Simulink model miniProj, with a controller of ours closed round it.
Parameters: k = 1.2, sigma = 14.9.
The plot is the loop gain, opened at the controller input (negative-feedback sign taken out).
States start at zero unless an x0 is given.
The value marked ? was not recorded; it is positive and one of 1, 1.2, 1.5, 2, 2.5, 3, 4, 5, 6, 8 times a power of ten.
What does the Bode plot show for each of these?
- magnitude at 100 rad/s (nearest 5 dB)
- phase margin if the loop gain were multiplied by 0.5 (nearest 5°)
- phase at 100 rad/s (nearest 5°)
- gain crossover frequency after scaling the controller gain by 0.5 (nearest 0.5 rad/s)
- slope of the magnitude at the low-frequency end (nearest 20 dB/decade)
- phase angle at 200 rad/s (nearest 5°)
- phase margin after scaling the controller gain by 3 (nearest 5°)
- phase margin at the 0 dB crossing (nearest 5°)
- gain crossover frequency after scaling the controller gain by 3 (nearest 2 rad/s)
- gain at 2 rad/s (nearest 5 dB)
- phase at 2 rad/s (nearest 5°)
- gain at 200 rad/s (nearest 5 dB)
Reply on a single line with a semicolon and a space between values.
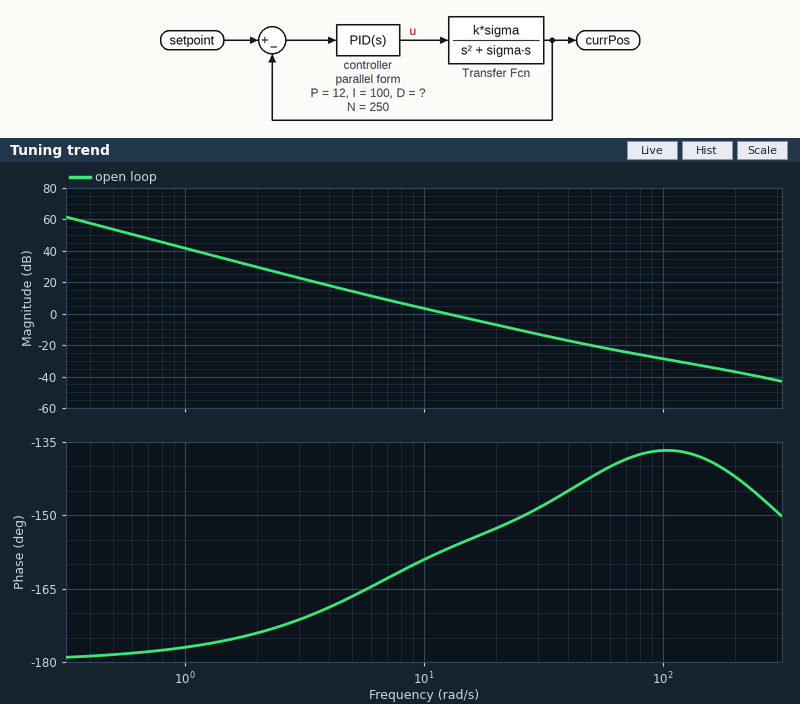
-30 dB; 20°; -135°; 8.5 rad/s; -40 dB/decade; -140°; 30°; 25°; 24 rad/s; 30 dB; -175°; -35 dB
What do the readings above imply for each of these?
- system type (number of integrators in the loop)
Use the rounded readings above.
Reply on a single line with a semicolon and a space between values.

2
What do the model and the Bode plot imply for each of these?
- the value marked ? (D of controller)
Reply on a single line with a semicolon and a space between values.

0.15
